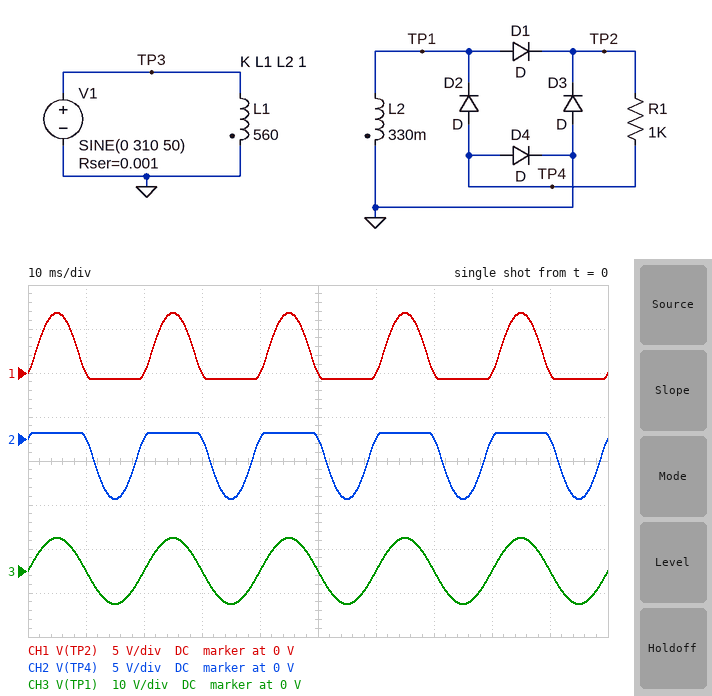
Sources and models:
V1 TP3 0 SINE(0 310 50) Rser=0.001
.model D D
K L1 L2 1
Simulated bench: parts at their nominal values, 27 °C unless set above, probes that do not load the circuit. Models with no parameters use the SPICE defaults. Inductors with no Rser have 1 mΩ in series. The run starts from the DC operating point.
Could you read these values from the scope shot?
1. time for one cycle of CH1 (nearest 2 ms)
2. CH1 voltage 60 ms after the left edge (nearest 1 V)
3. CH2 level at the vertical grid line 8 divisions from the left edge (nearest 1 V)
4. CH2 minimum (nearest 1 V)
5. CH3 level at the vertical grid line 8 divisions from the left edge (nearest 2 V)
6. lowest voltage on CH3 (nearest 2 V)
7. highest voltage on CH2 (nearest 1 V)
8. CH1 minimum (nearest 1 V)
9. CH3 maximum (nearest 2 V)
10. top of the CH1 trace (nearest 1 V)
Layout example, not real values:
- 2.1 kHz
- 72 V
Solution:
- 20 ms
- 0 V
- 0 V
- -7 V
- 0 V
- -8 V
- 1 V
- -1 V
- 8 V
- 7 V
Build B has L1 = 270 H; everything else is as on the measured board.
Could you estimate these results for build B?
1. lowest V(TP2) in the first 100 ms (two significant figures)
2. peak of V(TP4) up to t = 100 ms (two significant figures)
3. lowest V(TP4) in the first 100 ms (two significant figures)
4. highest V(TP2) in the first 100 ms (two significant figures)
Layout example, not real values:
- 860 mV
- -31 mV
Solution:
- -710 mV
- 710 mV
- -10 V
- 10 V
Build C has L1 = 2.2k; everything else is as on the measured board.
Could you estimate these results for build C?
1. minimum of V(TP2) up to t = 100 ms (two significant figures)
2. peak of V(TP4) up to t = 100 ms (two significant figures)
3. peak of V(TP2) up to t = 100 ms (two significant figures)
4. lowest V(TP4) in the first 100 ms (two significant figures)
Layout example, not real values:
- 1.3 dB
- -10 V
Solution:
- -680 mV
- 680 mV
- 3.1 V
- -3.1 V
